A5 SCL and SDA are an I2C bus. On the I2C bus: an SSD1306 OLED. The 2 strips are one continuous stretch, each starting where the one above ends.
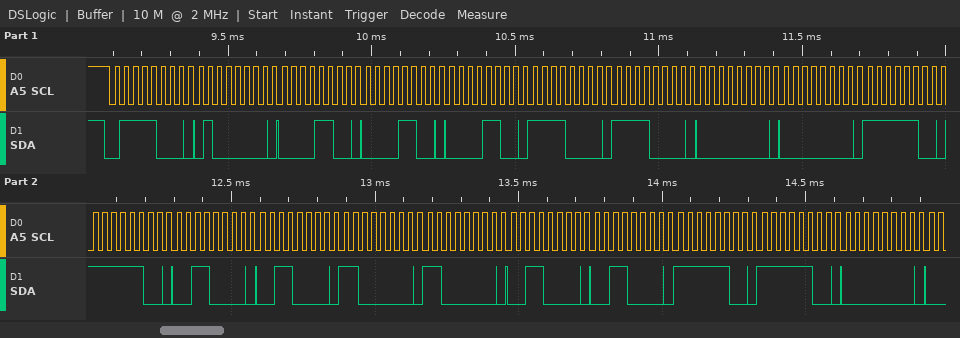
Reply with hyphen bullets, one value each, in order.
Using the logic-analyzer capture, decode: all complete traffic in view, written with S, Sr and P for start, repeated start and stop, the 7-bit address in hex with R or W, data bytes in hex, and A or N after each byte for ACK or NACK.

- S 3CW A 40 A 0C A 0C A 0C A F0 A F0 A 00 A 00 A FC A FC A 30 A 30 A C0 A C0 A 30 A 30 A FC A FC A 00 A
